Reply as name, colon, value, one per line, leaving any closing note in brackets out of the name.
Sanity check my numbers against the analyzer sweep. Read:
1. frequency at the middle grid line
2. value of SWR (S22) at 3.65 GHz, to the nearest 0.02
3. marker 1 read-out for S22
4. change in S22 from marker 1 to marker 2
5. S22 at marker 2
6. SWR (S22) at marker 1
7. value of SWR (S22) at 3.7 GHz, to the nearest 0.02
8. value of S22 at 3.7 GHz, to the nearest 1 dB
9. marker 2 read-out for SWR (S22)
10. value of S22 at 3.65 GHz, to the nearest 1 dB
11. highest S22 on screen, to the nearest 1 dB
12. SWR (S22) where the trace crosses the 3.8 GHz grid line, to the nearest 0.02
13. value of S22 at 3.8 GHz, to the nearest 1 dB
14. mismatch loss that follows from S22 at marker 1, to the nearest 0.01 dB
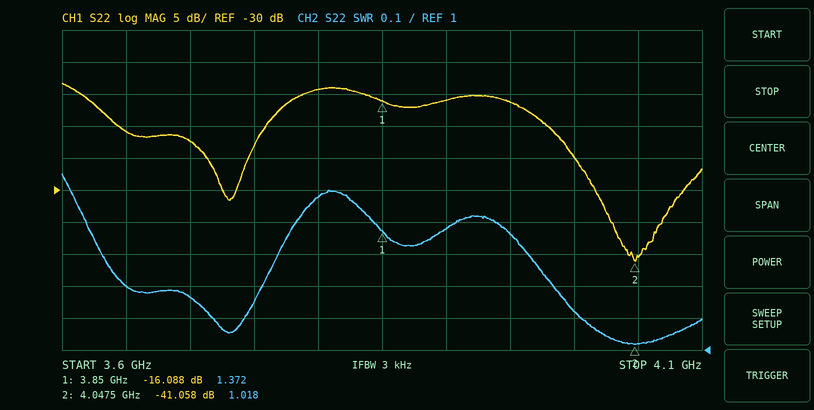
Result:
frequency at the middle grid line: 3.85 GHz
value of SWR (S22) at 3.65 GHz, to the nearest 0.02: 1.20
marker 1 read-out for S22: -16.088 dB
change in S22 from marker 1 to marker 2: -24.970 dB
S22 at marker 2: -41.058 dB
SWR (S22) at marker 1: 1.372
value of SWR (S22) at 3.7 GHz, to the nearest 0.02: 1.16
value of S22 at 3.7 GHz, to the nearest 1 dB: -22 dB
marker 2 read-out for SWR: 1.018
value of S22 at 3.65 GHz, to the nearest 1 dB: -21 dB
highest S22 on screen, to the nearest 1 dB: -13 dB
SWR (S22) where the trace crosses the 3.8 GHz grid line, to the nearest 0.02: 1.48
value of S22 at 3.8 GHz, to the nearest 1 dB: -14 dB
mismatch loss that follows from S22 at marker 1, to the nearest 0.01 dB: 0.11 dB
